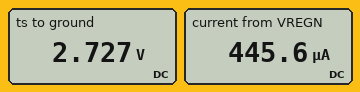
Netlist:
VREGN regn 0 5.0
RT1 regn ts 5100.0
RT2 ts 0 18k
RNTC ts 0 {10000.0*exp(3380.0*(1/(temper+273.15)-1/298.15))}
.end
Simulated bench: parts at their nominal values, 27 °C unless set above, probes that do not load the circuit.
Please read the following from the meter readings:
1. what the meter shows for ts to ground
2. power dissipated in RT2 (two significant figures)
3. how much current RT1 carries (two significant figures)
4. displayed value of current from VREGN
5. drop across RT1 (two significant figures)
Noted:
2.727 V
410 µW
450 µA
445.6 µA
2.3 V
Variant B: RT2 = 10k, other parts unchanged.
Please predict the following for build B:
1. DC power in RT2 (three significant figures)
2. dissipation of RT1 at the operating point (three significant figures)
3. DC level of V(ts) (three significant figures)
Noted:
589 µW
1.30 mW
2.43 V
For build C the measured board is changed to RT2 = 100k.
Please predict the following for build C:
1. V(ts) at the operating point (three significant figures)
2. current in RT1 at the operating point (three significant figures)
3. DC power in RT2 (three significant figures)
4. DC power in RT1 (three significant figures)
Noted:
3.12 V
368 µA
97.5 µW
691 µW
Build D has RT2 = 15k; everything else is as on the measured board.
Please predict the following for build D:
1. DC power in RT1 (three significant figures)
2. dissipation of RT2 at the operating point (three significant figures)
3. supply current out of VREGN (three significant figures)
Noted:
1.09 mW
467 µW
462 µA
